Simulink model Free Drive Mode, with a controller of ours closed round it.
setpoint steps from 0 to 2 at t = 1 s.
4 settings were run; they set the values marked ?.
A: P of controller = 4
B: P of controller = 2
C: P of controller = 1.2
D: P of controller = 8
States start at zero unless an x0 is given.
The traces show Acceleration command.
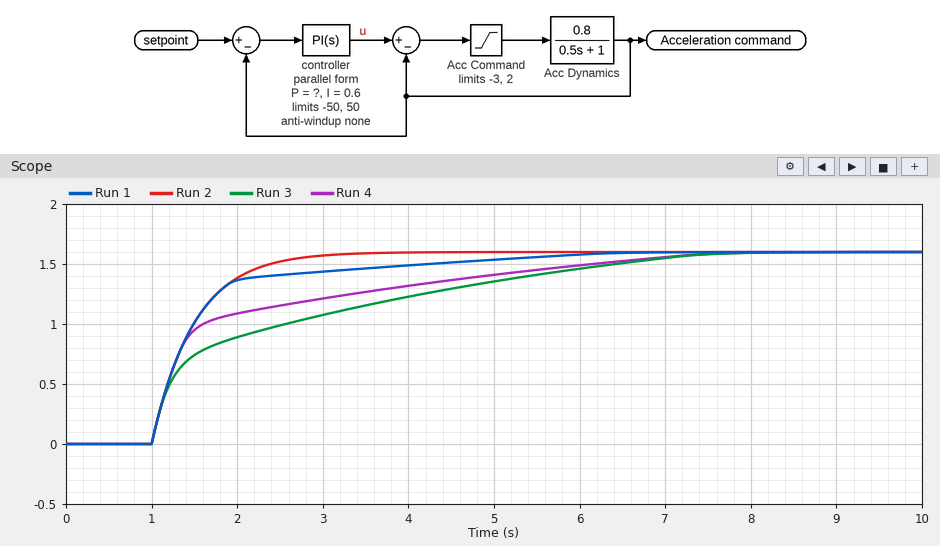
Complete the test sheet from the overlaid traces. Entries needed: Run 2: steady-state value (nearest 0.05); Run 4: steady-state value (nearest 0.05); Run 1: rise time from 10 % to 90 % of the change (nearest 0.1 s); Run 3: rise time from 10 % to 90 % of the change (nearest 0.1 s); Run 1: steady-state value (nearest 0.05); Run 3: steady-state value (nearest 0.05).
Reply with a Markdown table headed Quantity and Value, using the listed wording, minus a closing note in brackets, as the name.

| Quantity | Value |
|---|---|
| Run 2: steady-state value | 1.60 |
| Run 4: steady-state value | 1.60 |
| Run 1: rise time from 10 % to 90 % of the change | 2.0 s |
| Run 3: rise time from 10 % to 90 % of the change | 4.7 s |
| Run 1: steady-state value | 1.60 |
| Run 3: steady-state value | 1.60 |
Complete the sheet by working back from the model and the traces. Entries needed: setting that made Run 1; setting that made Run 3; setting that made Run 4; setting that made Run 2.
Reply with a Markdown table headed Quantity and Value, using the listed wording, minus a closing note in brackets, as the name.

| Quantity | Value |
|---|---|
| setting that made Run 1 | A |
| setting that made Run 3 | C |
| setting that made Run 4 | B |
| setting that made Run 2 | D |
